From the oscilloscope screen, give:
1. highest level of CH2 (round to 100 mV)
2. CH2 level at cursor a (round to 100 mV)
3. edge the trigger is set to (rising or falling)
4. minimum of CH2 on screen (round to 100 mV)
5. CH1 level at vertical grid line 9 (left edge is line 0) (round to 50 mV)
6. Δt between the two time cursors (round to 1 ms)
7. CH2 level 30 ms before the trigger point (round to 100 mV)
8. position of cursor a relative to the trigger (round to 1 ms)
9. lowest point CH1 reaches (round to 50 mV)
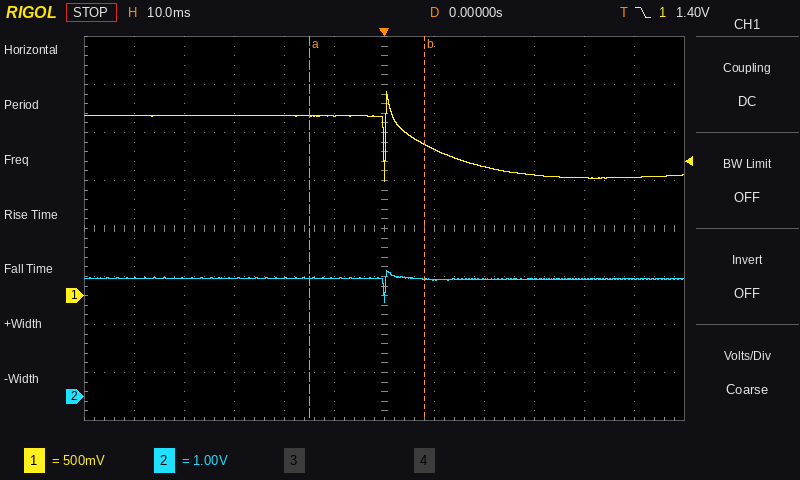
2.6 V
2.5 V
falling
2.0 V
1.25 V
23 ms
2.5 V
-15 ms
1.20 V
